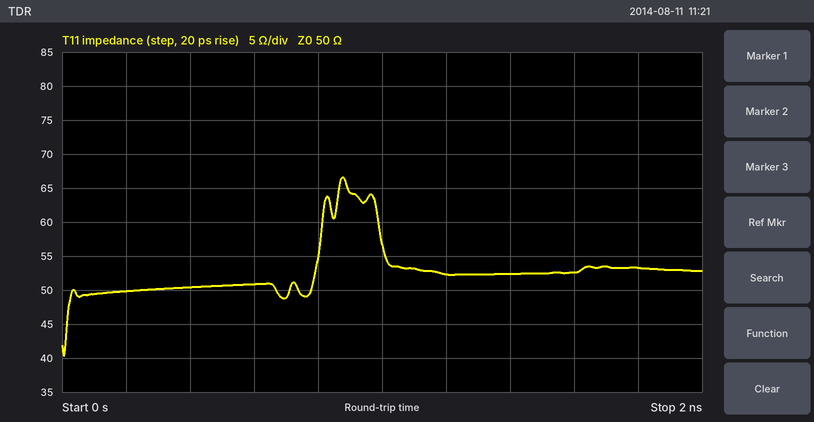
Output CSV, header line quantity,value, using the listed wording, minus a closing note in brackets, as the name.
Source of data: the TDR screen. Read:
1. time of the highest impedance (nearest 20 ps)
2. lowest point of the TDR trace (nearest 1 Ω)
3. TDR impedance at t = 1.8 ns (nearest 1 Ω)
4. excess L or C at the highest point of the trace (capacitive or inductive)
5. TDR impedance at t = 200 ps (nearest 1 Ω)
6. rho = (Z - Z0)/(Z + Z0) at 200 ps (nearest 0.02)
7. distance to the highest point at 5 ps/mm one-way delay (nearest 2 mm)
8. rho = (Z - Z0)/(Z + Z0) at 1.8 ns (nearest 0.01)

quantity,value
time of the highest impedance,880 ps
lowest point of the TDR trace,40 Ω
TDR impedance at t = 1.8 ns,53 Ω
excess L or C at the highest point of the trace,inductive
TDR impedance at t = 200 ps,50 Ω
rho = (Z - Z0)/(Z + Z0) at 200 ps,0.00
distance to the highest point at 5 ps/mm one-way delay,88 mm
rho = (Z - Z0)/(Z + Z0) at 1.8 ns,+0.03
